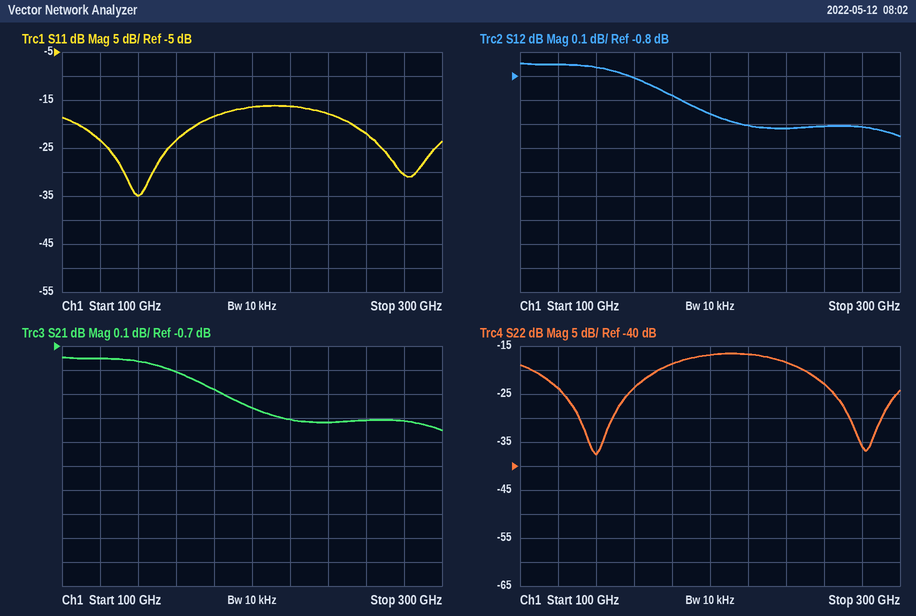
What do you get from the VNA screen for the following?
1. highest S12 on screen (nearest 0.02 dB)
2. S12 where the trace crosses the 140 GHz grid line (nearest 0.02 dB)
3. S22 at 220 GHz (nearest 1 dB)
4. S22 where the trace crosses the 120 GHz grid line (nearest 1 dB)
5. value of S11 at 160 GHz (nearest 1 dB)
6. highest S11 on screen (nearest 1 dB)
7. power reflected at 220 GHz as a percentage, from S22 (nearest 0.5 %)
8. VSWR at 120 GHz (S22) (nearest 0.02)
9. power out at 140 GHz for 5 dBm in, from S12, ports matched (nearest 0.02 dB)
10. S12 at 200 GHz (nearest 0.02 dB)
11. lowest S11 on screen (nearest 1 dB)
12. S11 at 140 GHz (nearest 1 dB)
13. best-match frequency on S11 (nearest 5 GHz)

-0.74 dB
-0.76 dB
-17 dB
-24 dB
-23 dB
-16 dB
2.0 %
1.14
4.24 dBm
-0.96 dB
-35 dB
-35 dB
140 GHz
